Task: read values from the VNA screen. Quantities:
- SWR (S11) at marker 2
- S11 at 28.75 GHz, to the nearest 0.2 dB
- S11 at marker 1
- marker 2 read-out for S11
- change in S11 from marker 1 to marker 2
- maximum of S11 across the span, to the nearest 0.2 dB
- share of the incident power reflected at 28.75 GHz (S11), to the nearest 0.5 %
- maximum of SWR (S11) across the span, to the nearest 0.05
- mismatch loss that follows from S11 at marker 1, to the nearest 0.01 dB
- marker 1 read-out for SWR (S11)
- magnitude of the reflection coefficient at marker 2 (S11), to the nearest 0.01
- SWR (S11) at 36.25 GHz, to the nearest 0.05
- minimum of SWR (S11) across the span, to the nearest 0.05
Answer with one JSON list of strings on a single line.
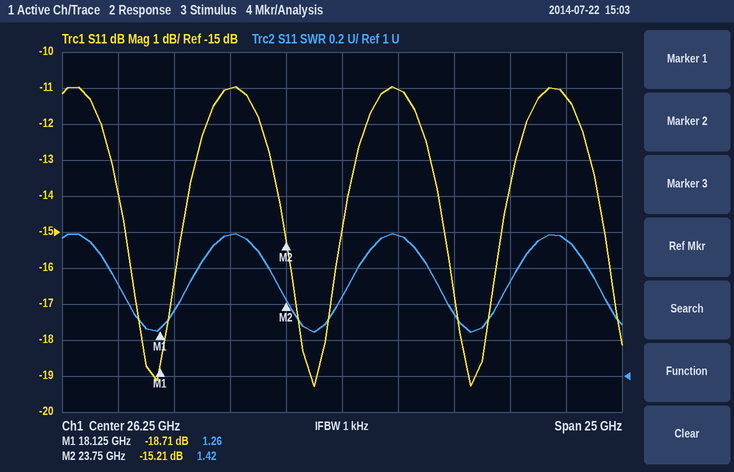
["1.42", "-11.0 dB", "-18.71 dB", "-15.21 dB", "3.50 dB", "-11.0 dB", "8.0 %", "1.80", "0.06 dB", "1.26", "0.17", "1.75", "1.25"]
